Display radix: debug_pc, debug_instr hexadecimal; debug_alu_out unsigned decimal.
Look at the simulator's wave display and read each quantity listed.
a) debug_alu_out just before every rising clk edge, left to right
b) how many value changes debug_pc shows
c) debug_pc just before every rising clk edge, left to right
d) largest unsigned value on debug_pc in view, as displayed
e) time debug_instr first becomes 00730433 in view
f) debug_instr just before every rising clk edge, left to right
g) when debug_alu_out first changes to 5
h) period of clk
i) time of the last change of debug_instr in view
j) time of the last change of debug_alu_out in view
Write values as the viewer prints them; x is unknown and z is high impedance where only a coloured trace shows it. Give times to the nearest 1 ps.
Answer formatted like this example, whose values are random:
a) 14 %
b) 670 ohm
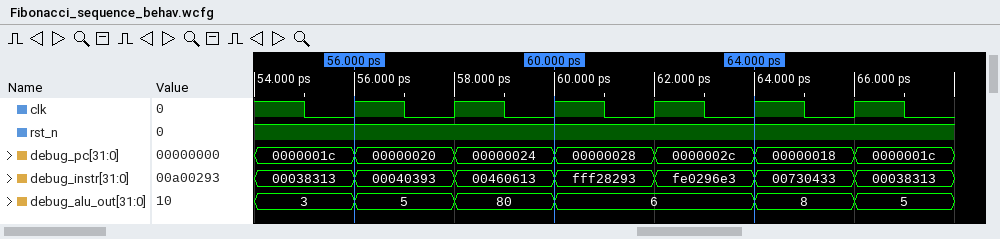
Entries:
a) 3, 5, 80, 6, 6, 8
b) 6
c) 0000001c, 00000020, 00000024, 00000028, 0000002c, 00000018
d) 0000002c
e) 64 ps
f) 00038313, 00040393, 00460613, fff28293, fe0296e3, 00730433
g) 56 ps
h) 2 ps
i) 66 ps
j) 66 ps
